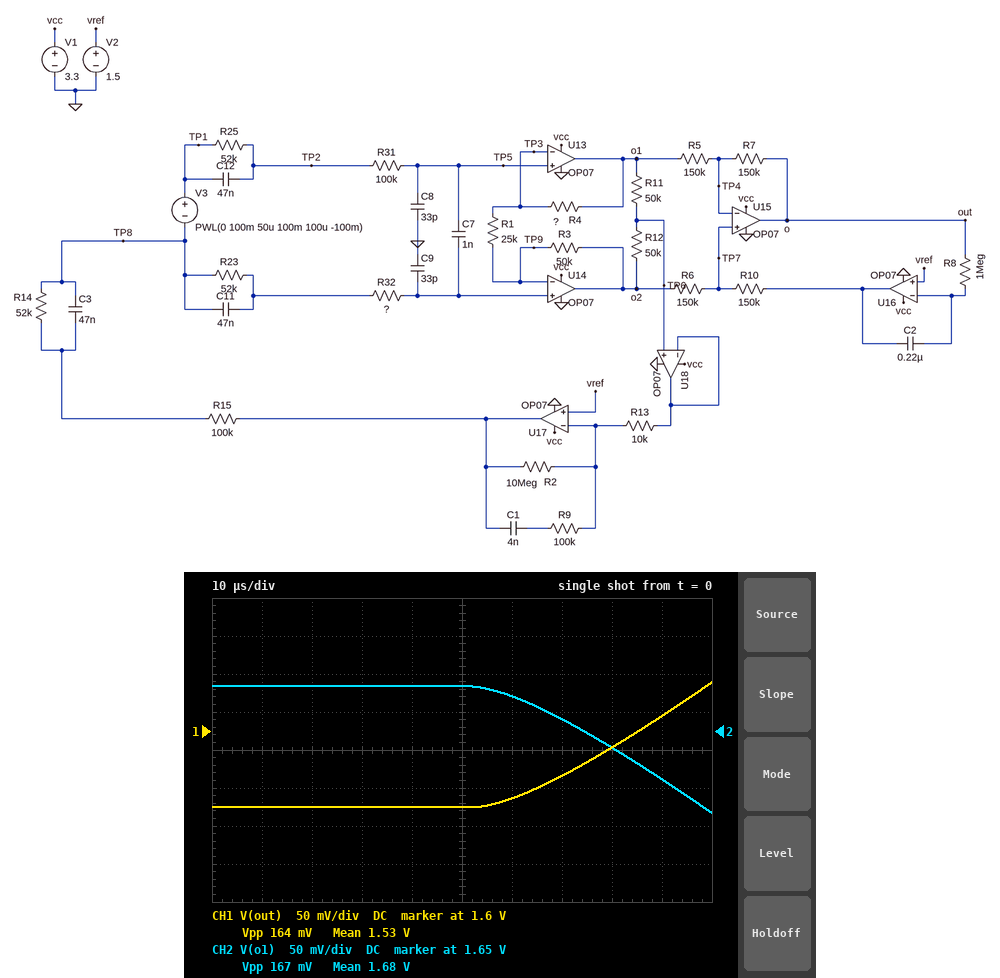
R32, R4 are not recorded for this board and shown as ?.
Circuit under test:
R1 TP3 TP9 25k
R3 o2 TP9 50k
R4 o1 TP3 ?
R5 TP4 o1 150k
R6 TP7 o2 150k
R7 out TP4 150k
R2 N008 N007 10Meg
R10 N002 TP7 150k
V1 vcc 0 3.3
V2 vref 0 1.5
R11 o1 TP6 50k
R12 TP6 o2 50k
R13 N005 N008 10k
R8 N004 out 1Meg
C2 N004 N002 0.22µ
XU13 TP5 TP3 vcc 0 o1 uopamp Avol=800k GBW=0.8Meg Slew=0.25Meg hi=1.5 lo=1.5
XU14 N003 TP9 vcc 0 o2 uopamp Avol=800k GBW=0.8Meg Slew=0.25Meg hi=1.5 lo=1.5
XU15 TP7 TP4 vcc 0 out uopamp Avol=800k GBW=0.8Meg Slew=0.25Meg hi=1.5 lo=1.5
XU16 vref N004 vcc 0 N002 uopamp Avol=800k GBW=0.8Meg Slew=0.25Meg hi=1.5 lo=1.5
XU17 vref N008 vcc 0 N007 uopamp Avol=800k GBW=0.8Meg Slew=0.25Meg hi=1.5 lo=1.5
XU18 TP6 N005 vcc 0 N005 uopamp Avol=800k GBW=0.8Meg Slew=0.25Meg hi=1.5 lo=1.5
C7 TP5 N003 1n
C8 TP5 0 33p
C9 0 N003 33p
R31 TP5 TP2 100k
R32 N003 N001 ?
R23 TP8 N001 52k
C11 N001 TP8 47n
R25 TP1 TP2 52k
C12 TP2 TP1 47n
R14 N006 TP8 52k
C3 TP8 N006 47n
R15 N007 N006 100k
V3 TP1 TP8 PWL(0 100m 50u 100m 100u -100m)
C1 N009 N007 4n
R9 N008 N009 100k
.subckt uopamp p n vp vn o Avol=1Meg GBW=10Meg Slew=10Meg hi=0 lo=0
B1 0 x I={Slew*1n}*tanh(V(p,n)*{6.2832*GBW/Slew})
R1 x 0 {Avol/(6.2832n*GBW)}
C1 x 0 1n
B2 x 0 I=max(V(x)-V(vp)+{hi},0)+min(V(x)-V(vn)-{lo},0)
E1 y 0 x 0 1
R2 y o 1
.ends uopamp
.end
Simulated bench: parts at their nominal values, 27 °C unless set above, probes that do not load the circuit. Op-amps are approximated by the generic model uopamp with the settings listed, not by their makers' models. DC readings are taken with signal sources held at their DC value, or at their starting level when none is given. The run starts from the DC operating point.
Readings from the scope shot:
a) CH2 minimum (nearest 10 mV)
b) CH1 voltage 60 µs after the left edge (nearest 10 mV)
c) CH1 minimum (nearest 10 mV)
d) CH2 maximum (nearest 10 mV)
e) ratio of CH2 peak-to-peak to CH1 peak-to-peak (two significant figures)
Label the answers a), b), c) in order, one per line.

a) 1.54 V
b) 1.51 V
c) 1.50 V
d) 1.71 V
e) 1.0
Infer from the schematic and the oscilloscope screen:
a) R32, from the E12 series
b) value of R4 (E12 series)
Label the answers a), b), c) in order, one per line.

a) 68 kΩ
b) 82 kΩ
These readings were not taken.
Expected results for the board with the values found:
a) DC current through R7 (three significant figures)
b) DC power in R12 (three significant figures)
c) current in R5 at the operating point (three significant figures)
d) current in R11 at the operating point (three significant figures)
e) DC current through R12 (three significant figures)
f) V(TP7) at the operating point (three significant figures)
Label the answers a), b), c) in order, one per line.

a) 697 nA
b) 219 nW
c) 697 nA
d) 2.09 µA
e) 2.09 µA
f) 1.60 V
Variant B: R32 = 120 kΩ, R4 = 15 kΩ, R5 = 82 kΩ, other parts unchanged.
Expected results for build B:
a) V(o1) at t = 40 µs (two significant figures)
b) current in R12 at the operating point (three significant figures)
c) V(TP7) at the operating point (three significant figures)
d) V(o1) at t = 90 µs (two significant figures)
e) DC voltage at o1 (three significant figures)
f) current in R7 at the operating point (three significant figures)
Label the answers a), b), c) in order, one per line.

a) 1.6 V
b) 1.20 µA
c) 1.58 V
d) 1.5 V
e) 1.62 V
f) 516 nA
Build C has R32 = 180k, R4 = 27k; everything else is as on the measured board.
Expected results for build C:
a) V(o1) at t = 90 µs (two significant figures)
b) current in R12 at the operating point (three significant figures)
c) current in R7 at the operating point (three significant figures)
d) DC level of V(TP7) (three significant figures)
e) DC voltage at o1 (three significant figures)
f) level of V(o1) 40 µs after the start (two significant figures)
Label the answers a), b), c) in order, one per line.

a) 1.5 V
b) 1.36 µA
c) 453 nA
d) 1.57 V
e) 1.64 V
f) 1.6 V
